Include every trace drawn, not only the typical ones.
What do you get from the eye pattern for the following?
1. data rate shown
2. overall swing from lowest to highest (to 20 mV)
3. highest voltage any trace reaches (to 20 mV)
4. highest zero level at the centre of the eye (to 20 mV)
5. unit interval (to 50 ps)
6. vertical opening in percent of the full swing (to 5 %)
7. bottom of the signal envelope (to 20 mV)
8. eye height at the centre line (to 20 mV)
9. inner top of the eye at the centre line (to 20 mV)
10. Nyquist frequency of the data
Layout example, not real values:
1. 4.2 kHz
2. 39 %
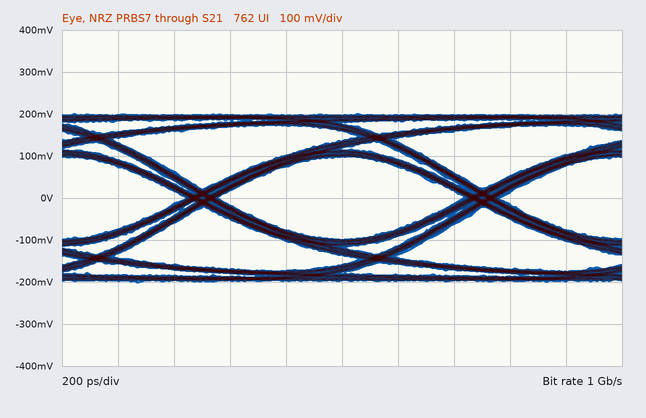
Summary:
1. 1 Gb/s
2. 400 mV
3. 200 mV
4. -100 mV
5. 1.00 ns
6. 50 %
7. -200 mV
8. 200 mV
9. 100 mV
10. 500 MHz
